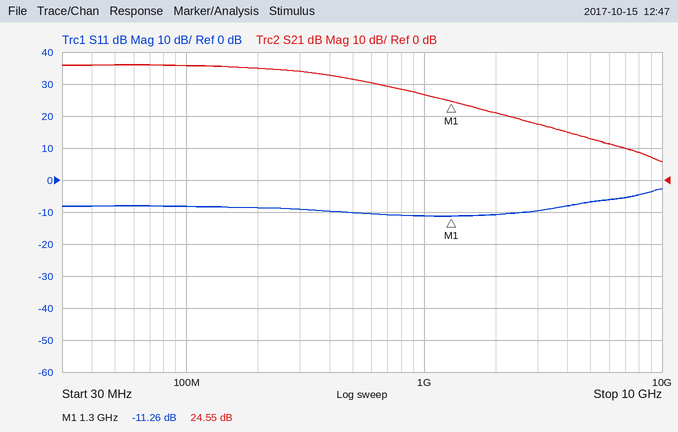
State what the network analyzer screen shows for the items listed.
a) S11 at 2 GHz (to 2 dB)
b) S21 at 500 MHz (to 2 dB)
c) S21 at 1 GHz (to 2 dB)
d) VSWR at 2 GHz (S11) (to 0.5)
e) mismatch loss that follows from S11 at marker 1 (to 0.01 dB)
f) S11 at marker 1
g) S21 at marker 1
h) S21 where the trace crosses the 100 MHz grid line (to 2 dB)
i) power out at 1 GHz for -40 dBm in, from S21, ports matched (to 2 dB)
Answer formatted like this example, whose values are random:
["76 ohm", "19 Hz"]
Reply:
["-10 dB", "32 dB", "26 dB", "2.0", "0.34 dB", "-11.26 dB", "24.55 dB", "36 dB", "-14 dBm"]
